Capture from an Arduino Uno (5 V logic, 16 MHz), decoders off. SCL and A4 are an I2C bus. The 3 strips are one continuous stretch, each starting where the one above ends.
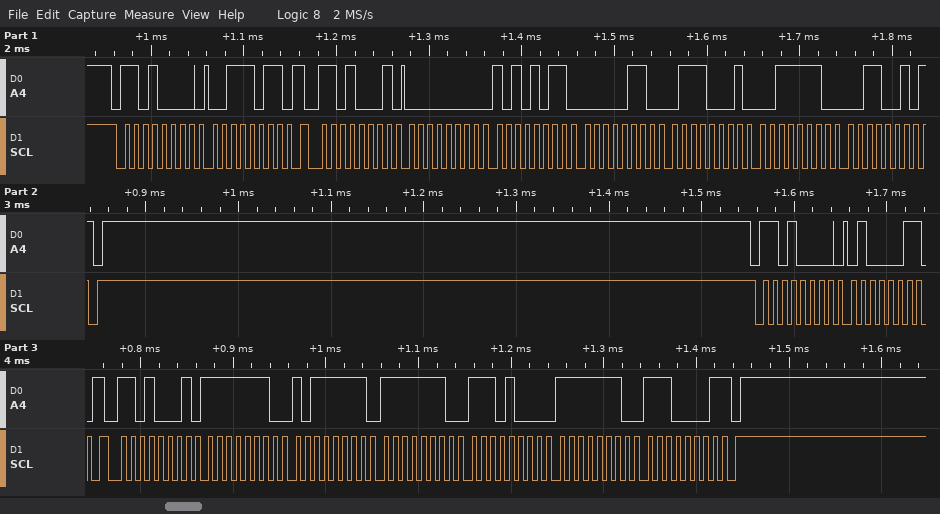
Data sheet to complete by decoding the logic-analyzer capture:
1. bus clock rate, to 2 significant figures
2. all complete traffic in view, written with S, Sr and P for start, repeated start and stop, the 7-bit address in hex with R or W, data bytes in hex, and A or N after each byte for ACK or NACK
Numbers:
100 kHz
S 68W A 3B A Sr 68R A 00 A AB A 06 A 71 A 3E A 32 N P S 68W A 43 A Sr 68R A FE A BF A FE A E8 A FE A E1 N P
